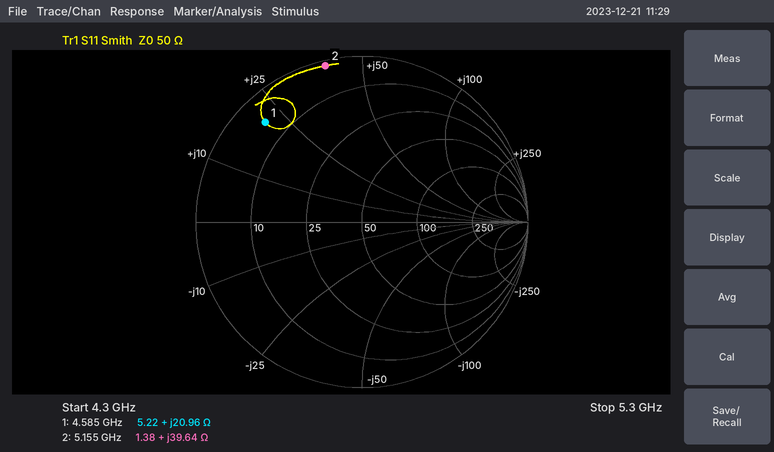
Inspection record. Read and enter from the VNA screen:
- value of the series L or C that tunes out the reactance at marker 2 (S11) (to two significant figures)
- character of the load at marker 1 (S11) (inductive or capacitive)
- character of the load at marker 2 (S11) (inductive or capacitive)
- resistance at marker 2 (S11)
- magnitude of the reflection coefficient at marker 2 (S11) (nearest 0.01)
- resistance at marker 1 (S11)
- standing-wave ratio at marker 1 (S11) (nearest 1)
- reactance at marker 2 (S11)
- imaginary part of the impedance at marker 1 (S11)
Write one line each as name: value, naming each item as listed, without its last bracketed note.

value of the series L or C that tunes out the reactance at marker 2 (S11): 780 fF
character of the load at marker 1 (S11): inductive
character of the load at marker 2 (S11): inductive
resistance at marker 2: 1.38 Ω
magnitude of the reflection coefficient at marker 2 (S11): 0.97
resistance at marker 1: 5.22 Ω
standing-wave ratio at marker 1 (S11): 11
reactance at marker 2: +39.64 Ω
imaginary part of the impedance at marker 1: +20.96 Ω
